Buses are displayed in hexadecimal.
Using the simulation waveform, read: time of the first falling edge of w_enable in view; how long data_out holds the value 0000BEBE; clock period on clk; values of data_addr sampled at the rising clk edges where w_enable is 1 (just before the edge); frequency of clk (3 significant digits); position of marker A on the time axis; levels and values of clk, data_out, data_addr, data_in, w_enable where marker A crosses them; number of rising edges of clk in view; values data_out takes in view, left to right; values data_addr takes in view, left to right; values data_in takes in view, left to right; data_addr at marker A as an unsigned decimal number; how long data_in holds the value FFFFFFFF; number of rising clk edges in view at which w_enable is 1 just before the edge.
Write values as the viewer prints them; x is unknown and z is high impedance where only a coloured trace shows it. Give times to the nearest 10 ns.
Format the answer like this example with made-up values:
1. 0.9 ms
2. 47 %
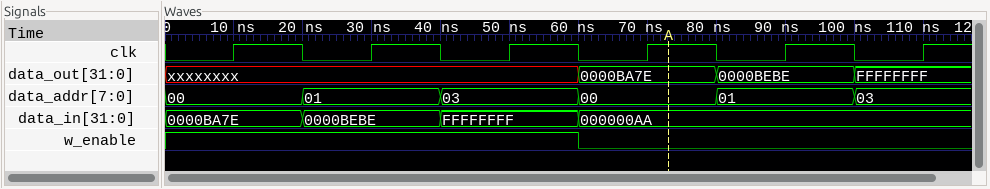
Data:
1. 60 ns
2. 20 ns
3. 20 ns
4. 00, 01, 03
5. 50.0 MHz
6. 70 ns
7. clk=1, data_out=0000BA7E, data_addr=00, data_in=000000AA, w_enable=0
8. 6
9. xxxxxxxx, 0000BA7E, 0000BEBE, FFFFFFFF
10. 00, 01, 03, 00, 01, 03
11. 0000BA7E, 0000BEBE, FFFFFFFF, 000000AA
12. 0
13. 20 ns
14. 3
